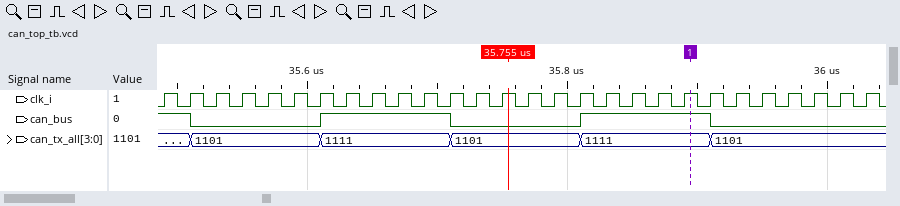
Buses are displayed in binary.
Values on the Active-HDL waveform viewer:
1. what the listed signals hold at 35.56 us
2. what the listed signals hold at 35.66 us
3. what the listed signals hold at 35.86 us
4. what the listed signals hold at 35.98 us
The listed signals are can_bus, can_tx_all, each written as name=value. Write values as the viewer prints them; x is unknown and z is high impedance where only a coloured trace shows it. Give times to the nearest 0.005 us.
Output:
can_bus=0, can_tx_all=1101
can_bus=1, can_tx_all=1111
can_bus=1, can_tx_all=1111
can_bus=0, can_tx_all=1101
